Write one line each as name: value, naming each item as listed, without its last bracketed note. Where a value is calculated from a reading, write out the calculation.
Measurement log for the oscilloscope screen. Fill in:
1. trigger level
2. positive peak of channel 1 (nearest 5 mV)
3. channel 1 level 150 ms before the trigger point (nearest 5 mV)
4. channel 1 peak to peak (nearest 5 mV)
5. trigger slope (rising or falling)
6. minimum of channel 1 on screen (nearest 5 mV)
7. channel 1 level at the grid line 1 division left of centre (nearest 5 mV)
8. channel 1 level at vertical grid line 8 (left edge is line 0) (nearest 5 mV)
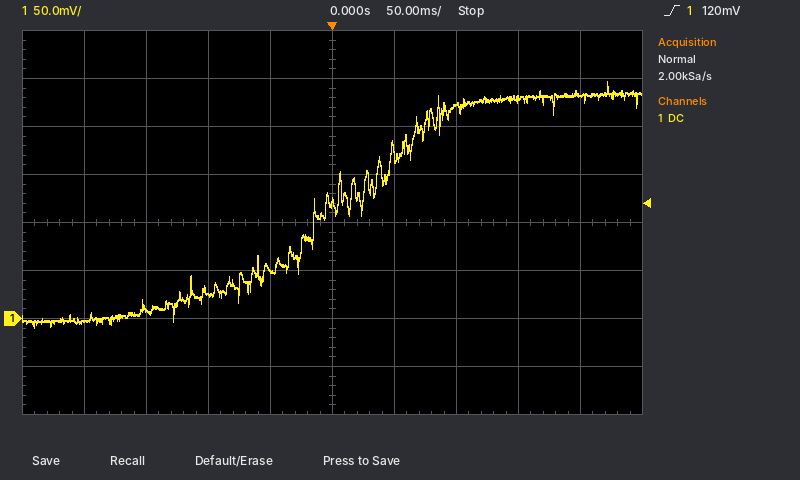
trigger level: 120 mV
positive peak of channel 1: 245 mV
channel 1 level 150 ms before the trigger point: 10 mV
channel 1 peak to peak: 245 mV − (-10 mV) = 255 mV
trigger slope: rising
minimum of channel 1 on screen: -10 mV
channel 1 level at the grid line 1 division left of centre: 50 mV
channel 1 level at vertical grid line 8 (left edge is line 0): 230 mV
